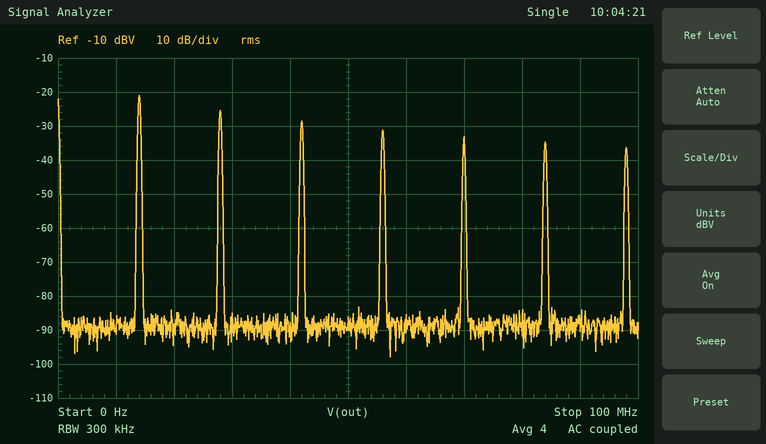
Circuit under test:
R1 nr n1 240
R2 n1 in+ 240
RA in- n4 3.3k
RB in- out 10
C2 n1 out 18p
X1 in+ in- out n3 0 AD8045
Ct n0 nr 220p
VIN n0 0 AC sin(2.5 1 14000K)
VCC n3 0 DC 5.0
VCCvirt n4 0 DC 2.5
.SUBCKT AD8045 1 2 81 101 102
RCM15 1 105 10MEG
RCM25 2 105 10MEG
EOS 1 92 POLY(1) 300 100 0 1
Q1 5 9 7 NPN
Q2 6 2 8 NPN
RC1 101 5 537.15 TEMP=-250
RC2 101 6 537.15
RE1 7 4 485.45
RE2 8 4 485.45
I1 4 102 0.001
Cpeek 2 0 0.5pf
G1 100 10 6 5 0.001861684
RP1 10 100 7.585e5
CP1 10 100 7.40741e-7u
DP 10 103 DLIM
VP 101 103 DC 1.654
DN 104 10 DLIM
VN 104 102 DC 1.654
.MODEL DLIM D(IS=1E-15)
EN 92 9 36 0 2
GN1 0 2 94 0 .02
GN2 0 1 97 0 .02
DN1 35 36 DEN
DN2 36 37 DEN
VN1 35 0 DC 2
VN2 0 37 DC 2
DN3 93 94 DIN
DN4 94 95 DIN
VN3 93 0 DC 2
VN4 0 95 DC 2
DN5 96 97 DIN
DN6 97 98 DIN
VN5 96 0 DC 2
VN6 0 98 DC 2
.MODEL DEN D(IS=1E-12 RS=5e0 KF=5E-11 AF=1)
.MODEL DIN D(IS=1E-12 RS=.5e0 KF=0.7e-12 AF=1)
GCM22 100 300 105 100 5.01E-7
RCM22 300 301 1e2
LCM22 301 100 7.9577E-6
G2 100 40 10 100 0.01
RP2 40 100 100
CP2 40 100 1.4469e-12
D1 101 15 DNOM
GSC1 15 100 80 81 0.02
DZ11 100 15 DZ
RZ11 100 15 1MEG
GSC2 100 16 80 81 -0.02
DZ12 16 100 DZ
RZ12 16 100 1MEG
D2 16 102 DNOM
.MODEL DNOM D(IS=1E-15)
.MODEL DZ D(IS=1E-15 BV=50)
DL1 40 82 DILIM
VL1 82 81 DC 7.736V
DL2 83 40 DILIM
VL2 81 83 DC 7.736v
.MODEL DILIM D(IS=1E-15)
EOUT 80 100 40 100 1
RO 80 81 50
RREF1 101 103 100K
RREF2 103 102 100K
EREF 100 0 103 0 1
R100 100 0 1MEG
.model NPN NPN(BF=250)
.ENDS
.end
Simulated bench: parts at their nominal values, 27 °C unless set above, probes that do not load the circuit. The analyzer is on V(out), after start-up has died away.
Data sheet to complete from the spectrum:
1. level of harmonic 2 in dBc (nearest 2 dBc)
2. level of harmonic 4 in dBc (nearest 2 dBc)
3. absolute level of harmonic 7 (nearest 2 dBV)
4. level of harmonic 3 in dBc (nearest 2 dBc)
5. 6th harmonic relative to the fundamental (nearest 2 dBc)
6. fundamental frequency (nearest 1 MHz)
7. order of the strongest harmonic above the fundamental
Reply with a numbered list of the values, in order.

1. -4 dBc
2. -10 dBc
3. -36 dBV
4. -8 dBc
5. -14 dBc
6. 14 MHz
7. 2
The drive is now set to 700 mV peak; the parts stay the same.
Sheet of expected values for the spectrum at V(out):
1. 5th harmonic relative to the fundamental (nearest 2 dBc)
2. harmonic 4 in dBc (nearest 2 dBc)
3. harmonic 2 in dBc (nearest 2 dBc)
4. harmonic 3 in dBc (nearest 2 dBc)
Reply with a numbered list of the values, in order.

1. -38 dBc
2. -32 dBc
3. -12 dBc
4. -20 dBc
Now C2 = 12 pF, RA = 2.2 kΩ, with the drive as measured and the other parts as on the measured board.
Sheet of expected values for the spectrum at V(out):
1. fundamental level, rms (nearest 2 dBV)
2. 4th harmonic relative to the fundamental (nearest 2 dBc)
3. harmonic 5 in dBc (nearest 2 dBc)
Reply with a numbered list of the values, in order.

1. -20 dBV
2. -12 dBc
3. -18 dBc
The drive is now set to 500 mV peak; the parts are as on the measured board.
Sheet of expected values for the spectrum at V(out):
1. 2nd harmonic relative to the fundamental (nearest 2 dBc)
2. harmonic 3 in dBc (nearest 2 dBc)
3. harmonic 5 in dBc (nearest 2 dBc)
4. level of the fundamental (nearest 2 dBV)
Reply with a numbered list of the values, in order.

1. -16 dBc
2. -28 dBc
3. -50 dBc
4. -32 dBV
